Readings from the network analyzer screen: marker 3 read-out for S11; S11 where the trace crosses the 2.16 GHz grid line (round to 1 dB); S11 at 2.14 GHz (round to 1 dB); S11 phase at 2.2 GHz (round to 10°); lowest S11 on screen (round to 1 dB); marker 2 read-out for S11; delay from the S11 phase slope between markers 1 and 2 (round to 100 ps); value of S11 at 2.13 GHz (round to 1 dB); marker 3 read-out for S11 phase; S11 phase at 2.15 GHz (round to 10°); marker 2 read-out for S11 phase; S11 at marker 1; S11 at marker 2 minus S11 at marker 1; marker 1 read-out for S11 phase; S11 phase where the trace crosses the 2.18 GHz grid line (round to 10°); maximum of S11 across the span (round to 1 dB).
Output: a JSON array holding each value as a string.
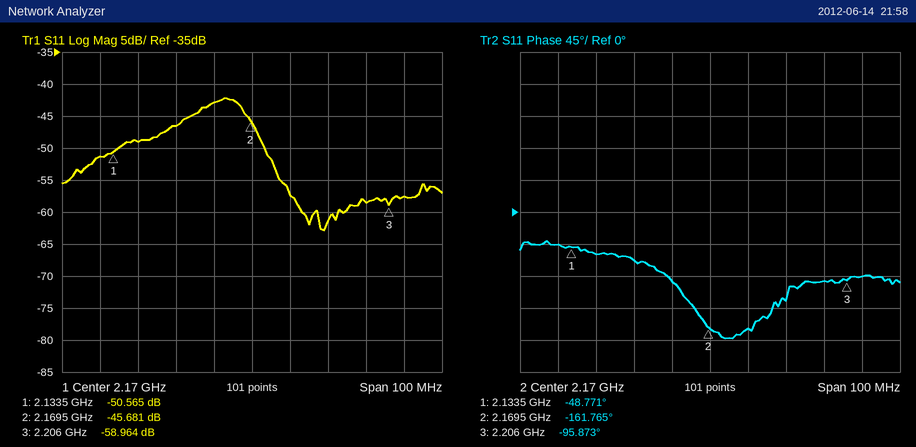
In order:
["-58.964 dB", "-43 dB", "-49 dB", "-100°", "-63 dB", "-45.681 dB", "8.7 ns", "-51 dB", "-95.873°", "-70°", "-161.765°", "-50.565 dB", "4.884 dB", "-48.771°", "-160°", "-42 dB"]
